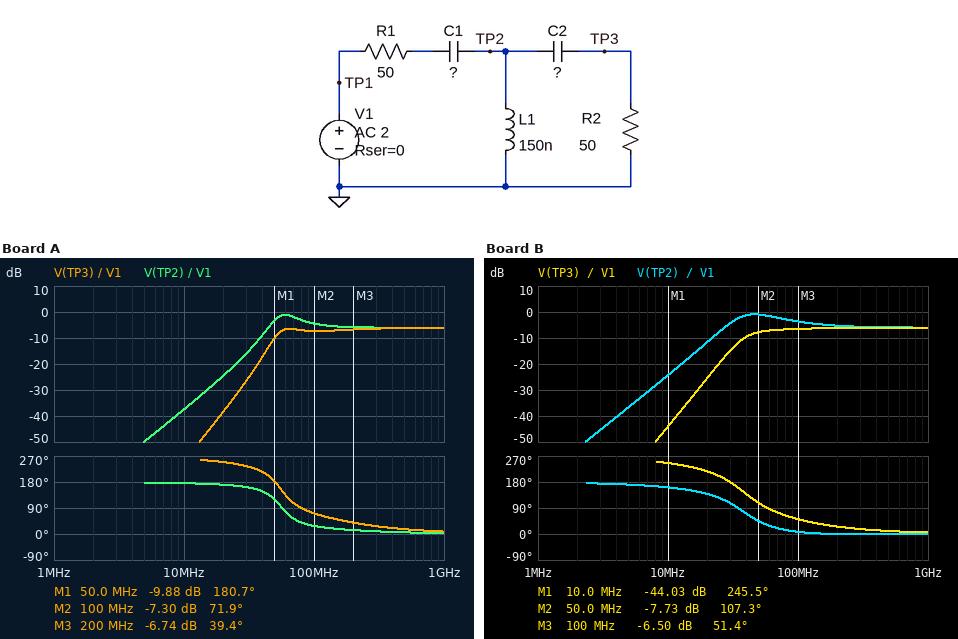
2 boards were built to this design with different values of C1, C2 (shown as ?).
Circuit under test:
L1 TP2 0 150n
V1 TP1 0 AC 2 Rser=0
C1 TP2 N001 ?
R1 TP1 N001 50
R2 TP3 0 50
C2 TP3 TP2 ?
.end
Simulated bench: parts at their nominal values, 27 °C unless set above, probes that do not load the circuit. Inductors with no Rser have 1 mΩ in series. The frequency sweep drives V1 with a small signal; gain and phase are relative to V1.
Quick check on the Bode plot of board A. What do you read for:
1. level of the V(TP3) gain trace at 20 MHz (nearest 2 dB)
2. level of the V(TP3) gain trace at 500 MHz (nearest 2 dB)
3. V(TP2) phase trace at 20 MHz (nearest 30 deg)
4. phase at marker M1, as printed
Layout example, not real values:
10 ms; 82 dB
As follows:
-38 dB; -6 dB; 180 deg; 180.7 deg
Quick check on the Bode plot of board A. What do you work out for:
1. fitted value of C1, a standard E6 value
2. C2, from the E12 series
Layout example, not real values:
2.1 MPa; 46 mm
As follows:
22 pF; 33 pF
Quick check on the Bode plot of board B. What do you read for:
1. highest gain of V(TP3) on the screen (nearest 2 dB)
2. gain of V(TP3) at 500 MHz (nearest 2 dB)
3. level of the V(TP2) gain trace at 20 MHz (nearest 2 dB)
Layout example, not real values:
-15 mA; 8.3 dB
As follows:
-6 dB; -6 dB; -12 dB
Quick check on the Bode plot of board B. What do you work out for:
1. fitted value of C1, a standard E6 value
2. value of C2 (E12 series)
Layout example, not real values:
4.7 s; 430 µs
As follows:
100 pF; 33 pF
